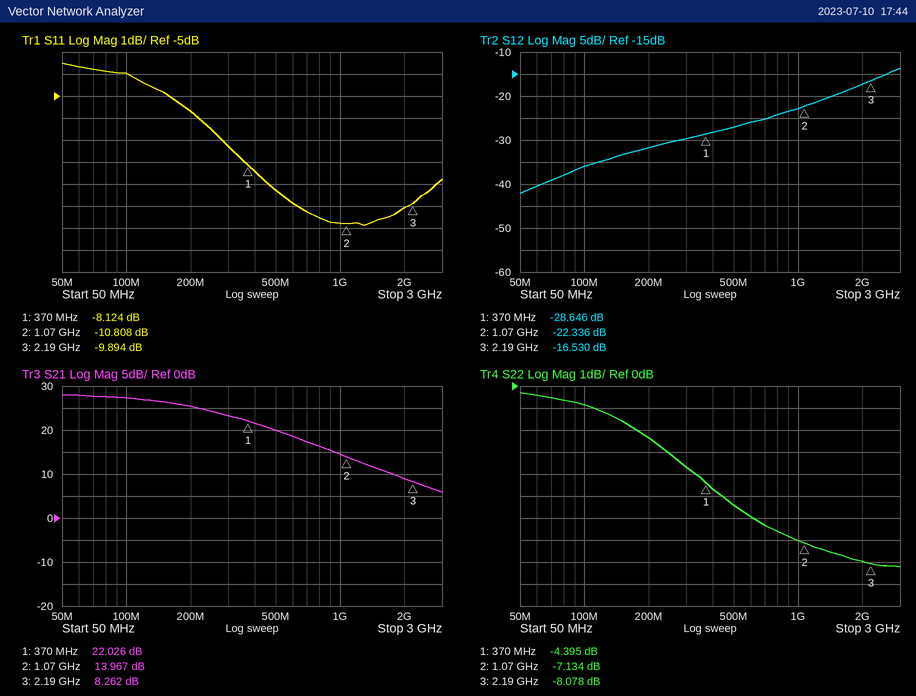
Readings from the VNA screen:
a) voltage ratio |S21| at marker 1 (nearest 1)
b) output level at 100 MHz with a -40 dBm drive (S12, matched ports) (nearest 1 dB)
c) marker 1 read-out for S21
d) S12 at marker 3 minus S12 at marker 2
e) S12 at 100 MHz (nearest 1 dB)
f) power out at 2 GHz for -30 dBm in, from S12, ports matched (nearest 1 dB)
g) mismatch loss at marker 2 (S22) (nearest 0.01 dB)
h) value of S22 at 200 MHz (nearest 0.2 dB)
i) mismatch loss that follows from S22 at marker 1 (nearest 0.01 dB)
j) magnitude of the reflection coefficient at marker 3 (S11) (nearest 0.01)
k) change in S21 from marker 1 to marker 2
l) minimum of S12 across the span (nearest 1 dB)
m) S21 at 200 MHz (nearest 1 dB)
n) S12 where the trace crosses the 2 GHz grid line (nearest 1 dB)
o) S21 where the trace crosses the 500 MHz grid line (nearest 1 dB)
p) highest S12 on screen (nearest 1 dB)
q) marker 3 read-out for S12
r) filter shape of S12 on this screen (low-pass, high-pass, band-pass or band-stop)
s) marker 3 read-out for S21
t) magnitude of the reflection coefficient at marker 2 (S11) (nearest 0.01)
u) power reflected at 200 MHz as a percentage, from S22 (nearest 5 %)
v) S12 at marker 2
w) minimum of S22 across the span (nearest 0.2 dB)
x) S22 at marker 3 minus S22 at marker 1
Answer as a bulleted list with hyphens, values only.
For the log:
- 13
- -76 dBm
- 22.026 dB
- 5.806 dB
- -36 dB
- -47 dBm
- 0.93 dB
- -2.4 dB
- 1.96 dB
- 0.32
- -8.059 dB
- -42 dB
- 25 dB
- -17 dB
- 20 dB
- -14 dB
- -16.530 dB
- high-pass
- 8.262 dB
- 0.29
- 60 %
- -22.336 dB
- -8.2 dB
- -3.683 dB
